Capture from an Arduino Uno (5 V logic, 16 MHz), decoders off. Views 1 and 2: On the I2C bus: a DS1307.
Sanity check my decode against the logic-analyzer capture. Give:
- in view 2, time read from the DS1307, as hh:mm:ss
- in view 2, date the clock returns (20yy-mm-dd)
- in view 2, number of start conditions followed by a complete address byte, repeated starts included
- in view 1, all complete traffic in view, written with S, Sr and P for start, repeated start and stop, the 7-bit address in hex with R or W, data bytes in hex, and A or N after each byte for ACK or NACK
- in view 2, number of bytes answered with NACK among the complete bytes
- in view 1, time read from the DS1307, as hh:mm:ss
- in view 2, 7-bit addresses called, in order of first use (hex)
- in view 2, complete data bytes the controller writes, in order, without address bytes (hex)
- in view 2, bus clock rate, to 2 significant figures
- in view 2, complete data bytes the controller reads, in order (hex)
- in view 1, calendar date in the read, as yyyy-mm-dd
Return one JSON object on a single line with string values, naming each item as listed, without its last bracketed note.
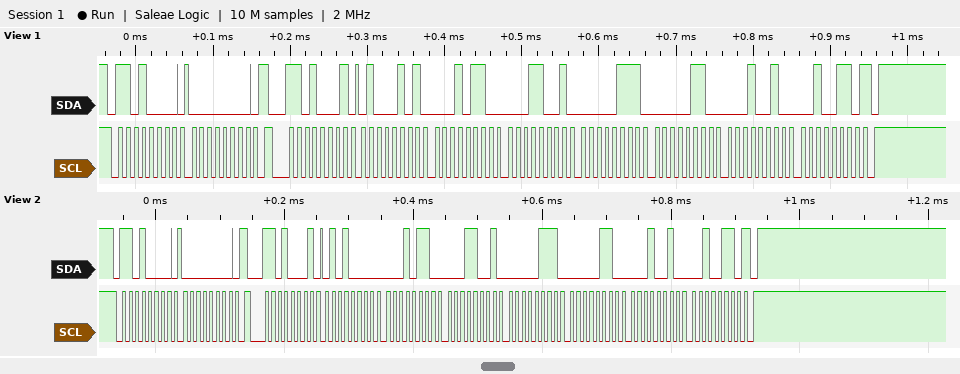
{"in view 2, time read from the DS1307, as hh:mm:ss": "19:16:50", "in view 2, date the clock returns": "2026-12-06", "in view 2, number of start conditions followed by a complete address byte, repeated starts included": "2", "in view 1, all complete traffic in view, written with S, Sr and P for start, repeated start and stop, the 7-bit address in hex with R or W, data bytes in hex, and A or N after each byte for ACK or NACK": "S 68W A 00 A Sr 68R A 45 A 16 A 19 A 07 A 06 A 12 A 26 N P", "in view 2, number of bytes answered with NACK among the complete bytes": "1", "in view 1, time read from the DS1307, as hh:mm:ss": "19:16:45", "in view 2, 7-bit addresses called, in order of first use": "0x68", "in view 2, complete data bytes the controller writes, in order, without address bytes": "00", "in view 2, bus clock rate, to 2 significant figures": "100 kHz", "in view 2, complete data bytes the controller reads, in order": "50 16 19 07 06 12 26", "in view 1, calendar date in the read, as yyyy-mm-dd": "2026-12-06"}
